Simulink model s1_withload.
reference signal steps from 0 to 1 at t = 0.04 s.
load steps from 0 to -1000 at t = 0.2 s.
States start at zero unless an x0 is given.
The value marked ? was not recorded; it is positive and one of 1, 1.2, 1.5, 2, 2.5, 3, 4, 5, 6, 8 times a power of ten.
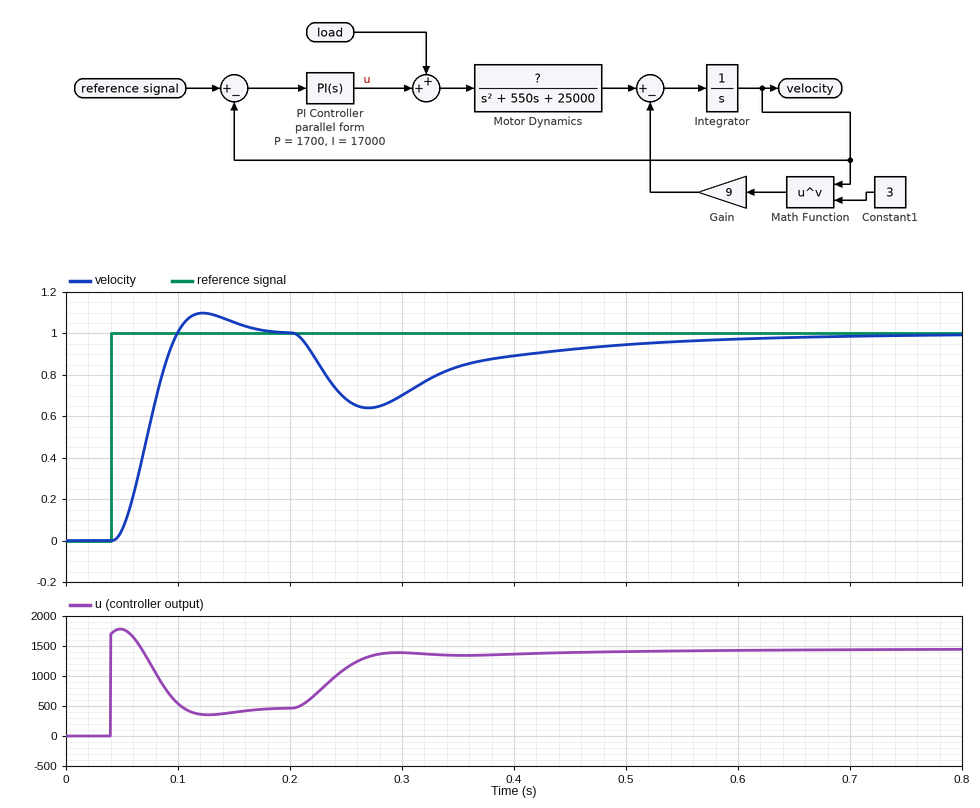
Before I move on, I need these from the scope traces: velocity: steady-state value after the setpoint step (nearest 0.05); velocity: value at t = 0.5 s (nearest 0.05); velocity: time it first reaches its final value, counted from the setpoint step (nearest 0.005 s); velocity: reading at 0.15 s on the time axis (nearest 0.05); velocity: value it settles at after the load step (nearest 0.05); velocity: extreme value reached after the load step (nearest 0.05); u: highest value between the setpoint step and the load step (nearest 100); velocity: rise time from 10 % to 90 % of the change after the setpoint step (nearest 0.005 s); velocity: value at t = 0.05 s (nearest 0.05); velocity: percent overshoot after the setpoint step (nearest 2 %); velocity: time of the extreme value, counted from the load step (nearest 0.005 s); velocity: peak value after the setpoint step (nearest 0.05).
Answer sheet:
1.00
0.95
0.060 s
1.05
1.00
0.65
1800
0.040 s
0.05
10 %
0.070 s
1.10
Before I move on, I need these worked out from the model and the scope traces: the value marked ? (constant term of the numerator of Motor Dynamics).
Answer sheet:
500
